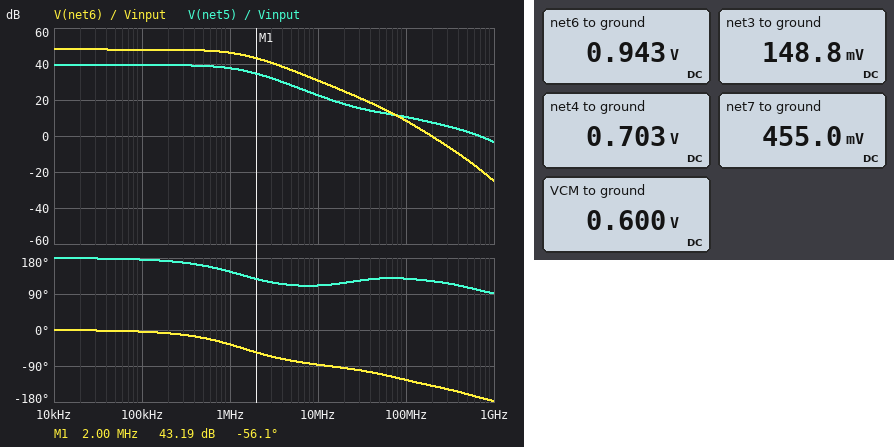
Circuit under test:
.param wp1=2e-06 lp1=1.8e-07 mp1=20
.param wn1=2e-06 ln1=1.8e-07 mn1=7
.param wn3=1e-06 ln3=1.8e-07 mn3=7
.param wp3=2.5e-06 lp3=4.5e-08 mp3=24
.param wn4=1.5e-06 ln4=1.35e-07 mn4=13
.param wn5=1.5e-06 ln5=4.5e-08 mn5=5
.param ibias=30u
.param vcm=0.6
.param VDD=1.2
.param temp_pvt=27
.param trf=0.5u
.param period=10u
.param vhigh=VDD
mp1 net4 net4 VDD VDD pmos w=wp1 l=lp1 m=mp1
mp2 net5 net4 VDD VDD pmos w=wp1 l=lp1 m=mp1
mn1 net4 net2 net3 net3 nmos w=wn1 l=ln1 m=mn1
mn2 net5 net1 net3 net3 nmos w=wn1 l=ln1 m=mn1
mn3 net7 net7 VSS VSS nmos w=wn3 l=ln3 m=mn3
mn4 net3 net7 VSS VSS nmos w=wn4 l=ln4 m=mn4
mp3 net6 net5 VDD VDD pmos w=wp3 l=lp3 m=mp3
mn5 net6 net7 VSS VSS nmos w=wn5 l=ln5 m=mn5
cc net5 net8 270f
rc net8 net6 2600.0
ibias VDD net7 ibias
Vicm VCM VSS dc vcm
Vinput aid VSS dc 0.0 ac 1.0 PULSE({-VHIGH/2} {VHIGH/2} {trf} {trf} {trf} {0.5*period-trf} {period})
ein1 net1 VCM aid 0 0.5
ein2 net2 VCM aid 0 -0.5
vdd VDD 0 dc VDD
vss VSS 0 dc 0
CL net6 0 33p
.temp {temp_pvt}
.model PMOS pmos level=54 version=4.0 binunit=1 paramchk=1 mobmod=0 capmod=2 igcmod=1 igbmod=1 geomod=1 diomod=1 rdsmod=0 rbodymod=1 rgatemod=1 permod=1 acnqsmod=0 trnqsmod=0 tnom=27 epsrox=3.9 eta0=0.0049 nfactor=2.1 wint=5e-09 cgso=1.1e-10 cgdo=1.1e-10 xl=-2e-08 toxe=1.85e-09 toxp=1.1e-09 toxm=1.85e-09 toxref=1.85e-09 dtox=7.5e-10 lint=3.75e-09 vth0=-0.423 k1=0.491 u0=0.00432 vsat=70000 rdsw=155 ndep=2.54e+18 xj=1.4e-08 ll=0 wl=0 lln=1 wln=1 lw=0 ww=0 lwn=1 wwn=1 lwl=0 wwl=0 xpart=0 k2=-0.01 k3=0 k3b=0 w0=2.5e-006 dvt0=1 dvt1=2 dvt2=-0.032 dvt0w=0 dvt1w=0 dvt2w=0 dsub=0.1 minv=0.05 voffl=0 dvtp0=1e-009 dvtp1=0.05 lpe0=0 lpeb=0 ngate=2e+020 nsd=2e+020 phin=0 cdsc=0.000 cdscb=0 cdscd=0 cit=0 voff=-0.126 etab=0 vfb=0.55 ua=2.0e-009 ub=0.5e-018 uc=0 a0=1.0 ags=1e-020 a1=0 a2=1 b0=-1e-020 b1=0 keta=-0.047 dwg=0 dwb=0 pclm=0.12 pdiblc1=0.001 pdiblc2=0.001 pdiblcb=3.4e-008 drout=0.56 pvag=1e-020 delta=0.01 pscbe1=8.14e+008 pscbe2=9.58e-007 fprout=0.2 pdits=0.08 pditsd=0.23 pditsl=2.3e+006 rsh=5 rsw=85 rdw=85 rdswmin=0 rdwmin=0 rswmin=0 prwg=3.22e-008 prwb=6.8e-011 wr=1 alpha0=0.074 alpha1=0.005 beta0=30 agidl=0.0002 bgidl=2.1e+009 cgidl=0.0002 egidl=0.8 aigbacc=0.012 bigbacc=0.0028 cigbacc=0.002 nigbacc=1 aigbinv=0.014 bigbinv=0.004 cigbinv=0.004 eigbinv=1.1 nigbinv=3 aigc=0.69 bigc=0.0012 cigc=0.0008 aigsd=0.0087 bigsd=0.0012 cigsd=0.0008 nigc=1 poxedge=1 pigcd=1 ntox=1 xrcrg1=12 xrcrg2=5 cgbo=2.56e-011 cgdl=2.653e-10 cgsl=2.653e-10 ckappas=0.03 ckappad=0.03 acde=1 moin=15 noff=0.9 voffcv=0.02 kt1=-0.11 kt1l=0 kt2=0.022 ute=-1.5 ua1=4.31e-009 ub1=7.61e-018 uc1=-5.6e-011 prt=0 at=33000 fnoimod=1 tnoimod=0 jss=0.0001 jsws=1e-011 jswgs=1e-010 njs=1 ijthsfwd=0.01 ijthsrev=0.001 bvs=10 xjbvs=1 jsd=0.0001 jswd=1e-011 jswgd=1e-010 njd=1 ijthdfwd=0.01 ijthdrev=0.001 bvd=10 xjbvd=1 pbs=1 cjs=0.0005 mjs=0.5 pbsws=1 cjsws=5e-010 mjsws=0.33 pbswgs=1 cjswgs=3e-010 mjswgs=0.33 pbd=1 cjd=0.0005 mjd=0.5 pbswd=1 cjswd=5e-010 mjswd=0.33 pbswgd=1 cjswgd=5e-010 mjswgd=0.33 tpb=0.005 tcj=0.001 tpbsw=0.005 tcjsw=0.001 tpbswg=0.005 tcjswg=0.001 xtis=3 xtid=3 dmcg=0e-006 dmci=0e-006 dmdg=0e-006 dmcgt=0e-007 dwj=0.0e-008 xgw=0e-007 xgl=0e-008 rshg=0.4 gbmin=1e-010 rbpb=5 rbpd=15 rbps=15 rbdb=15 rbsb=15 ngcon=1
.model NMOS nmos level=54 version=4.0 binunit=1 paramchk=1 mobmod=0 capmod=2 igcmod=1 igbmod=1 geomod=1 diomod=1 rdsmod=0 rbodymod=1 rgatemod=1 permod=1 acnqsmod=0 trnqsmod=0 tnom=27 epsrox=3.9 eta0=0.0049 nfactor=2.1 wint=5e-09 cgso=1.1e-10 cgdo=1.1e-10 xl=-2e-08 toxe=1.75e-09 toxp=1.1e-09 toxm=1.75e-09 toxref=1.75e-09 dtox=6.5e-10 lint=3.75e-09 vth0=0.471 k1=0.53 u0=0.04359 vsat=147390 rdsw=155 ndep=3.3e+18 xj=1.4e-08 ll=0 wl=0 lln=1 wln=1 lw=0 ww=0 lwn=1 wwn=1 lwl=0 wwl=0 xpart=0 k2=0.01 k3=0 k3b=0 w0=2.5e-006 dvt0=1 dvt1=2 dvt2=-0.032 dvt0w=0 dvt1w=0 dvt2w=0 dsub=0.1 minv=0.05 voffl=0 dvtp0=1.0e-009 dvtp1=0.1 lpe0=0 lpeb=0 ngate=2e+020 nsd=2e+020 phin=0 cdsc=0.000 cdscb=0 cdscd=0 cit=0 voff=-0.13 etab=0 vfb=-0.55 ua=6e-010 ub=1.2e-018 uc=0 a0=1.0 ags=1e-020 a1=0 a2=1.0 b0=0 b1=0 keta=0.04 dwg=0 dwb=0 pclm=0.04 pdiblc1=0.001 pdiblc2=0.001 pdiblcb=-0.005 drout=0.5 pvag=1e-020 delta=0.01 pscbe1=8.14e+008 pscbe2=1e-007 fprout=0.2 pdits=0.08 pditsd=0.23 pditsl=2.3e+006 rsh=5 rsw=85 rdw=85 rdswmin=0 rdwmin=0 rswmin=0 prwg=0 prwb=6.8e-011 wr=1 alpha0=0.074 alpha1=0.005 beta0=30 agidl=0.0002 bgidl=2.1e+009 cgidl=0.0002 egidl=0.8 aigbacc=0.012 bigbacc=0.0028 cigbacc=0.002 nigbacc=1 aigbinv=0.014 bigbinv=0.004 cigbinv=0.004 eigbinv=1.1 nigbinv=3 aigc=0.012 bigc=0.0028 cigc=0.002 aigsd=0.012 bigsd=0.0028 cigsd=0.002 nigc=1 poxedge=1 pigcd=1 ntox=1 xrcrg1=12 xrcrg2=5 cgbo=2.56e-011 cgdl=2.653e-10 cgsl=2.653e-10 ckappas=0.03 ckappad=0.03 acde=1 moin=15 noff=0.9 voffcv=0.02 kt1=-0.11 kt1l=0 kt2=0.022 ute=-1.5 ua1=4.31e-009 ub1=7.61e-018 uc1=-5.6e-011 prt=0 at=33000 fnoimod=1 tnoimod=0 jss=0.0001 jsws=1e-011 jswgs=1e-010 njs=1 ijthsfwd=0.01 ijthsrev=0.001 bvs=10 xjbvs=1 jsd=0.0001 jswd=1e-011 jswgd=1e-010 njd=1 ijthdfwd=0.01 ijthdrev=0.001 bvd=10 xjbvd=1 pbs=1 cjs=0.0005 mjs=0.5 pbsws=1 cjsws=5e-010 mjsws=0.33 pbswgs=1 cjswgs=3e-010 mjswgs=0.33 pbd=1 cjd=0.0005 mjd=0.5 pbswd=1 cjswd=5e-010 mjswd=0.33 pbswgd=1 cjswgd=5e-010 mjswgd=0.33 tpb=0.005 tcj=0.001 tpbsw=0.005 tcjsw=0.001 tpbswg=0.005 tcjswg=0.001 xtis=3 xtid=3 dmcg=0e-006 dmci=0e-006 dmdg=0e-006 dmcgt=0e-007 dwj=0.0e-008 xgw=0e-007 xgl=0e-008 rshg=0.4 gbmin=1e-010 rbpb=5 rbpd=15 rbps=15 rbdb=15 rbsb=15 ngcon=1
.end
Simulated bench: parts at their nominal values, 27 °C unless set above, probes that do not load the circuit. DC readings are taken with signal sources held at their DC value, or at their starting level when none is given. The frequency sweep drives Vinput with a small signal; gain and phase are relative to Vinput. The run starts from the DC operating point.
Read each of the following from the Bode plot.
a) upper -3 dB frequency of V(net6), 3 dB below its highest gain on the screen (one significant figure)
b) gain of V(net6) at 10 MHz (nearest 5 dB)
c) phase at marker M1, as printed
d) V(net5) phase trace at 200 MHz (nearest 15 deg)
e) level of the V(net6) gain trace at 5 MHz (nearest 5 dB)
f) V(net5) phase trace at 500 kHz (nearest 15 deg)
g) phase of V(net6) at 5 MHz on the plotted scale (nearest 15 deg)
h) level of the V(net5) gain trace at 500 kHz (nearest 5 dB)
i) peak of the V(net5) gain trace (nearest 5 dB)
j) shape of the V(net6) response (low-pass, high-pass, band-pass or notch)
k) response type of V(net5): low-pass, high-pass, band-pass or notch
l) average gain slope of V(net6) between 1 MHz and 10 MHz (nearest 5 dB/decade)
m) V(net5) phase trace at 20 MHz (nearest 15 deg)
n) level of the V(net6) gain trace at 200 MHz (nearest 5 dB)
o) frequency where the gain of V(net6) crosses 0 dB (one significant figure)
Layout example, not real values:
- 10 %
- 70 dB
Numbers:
- 1 MHz
- 30 dB
- -56.1 deg
- 120 deg
- 35 dB
- 165 deg
- -75 deg
- 40 dB
- 40 dB
- low-pass
- low-pass
- -15 dB/decade
- 120 deg
- 0 dB
- 200 MHz
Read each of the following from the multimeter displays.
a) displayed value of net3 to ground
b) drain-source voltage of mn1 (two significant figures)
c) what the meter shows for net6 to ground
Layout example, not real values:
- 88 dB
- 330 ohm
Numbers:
- 148.8 mV
- 550 mV
- 0.943 V
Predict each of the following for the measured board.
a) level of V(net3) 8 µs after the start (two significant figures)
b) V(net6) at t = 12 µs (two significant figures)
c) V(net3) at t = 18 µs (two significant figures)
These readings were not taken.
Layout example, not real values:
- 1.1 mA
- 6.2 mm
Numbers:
- 400 mV
- 1.2 V
- 400 mV
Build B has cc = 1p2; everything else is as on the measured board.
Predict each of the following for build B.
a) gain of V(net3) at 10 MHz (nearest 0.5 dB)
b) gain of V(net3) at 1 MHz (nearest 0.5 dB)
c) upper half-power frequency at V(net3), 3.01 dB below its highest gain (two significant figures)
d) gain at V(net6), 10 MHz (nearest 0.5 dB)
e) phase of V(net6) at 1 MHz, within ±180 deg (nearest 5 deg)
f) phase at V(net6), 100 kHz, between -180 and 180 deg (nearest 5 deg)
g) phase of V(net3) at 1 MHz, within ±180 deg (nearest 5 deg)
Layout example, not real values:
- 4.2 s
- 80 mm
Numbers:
- -40.5 dB
- -21.5 dB
- 370 kHz
- 19.5 dB
- -70 deg
- -15 deg
- 115 deg
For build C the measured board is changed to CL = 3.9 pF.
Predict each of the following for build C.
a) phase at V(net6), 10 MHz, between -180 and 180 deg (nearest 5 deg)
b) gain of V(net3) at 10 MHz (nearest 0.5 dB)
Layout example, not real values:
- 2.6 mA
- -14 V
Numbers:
- -80 deg
- -29.0 dB
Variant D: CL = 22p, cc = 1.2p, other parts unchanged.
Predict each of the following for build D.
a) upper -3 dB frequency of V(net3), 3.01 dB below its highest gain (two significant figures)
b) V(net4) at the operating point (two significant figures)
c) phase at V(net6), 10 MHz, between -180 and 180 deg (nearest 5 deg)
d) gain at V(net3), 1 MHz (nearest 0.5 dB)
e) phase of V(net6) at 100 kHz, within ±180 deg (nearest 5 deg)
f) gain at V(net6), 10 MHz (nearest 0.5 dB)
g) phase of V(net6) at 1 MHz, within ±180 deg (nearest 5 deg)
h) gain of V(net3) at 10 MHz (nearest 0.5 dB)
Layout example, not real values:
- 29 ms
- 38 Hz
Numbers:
- 370 kHz
- 700 mV
- -80 deg
- -21.5 dB
- -15 deg
- 19.5 dB
- -70 deg
- -40.5 dB
